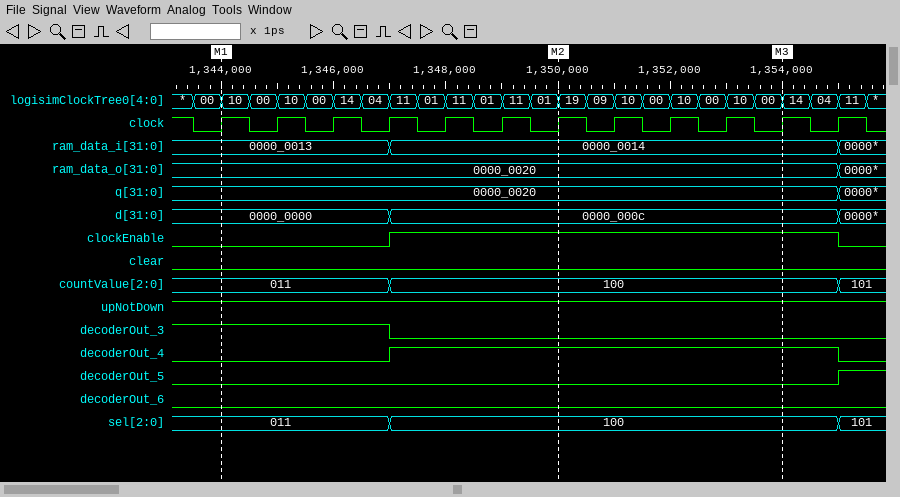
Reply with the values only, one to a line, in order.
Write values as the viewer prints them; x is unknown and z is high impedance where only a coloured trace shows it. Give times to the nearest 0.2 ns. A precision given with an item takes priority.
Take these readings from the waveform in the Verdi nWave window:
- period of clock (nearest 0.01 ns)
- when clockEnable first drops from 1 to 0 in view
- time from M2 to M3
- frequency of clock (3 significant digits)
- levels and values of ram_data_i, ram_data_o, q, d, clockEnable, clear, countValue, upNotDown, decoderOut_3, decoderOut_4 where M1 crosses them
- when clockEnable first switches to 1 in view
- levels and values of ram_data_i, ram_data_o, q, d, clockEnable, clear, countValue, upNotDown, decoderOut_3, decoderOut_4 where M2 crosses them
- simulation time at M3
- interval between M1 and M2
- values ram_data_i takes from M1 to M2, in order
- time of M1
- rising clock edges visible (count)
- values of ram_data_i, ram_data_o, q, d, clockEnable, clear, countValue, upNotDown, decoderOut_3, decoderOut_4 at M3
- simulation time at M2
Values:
1 ns
1355 ns
4 ns
1.00 GHz
ram_data_i=0000_0013, ram_data_o=0000_0020, q=0000_0020, d=0000_0000, clockEnable=0, clear=0, countValue=011, upNotDown=1, decoderOut_3=1, decoderOut_4=0
1347 ns
ram_data_i=0000_0014, ram_data_o=0000_0020, q=0000_0020, d=0000_000c, clockEnable=1, clear=0, countValue=100, upNotDown=1, decoderOut_3=0, decoderOut_4=1
1354 ns
6 ns
0000_0013, 0000_0014
1344 ns
12
ram_data_i=0000_0014, ram_data_o=0000_0020, q=0000_0020, d=0000_000c, clockEnable=1, clear=0, countValue=100, upNotDown=1, decoderOut_3=0, decoderOut_4=1
1350 ns
